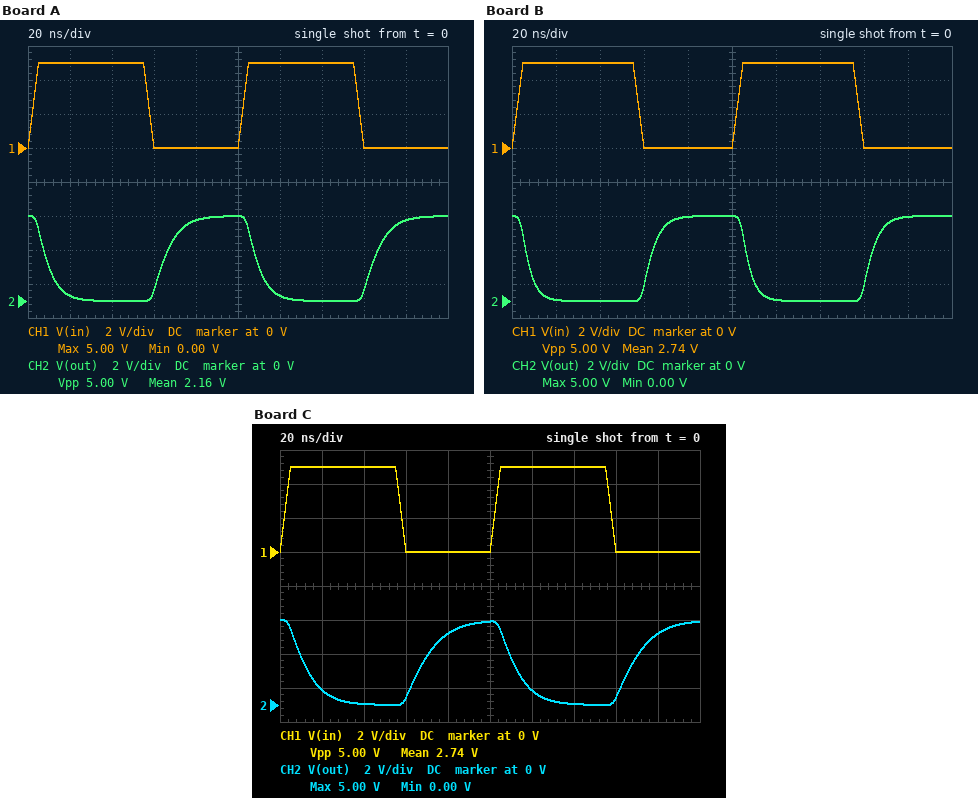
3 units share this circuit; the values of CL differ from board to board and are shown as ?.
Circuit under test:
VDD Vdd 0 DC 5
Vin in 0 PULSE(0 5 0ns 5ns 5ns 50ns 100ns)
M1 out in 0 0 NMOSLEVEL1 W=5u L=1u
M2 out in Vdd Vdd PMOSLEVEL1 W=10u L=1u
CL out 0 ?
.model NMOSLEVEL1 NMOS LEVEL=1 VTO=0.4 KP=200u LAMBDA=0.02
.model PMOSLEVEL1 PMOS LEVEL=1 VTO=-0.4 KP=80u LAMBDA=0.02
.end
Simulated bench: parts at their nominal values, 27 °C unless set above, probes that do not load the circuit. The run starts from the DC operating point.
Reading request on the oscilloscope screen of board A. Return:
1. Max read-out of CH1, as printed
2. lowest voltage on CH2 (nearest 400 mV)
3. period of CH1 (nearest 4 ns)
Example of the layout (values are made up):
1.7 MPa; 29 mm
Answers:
5.00 V; 0 V; 100 ns
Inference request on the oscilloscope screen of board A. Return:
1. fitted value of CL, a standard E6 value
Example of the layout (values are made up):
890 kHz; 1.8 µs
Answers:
22 pF
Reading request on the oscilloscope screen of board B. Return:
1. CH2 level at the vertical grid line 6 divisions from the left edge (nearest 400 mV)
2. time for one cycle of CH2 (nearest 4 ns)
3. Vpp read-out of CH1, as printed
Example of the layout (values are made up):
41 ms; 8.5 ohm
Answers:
0 V; 100 ns; 5.00 V
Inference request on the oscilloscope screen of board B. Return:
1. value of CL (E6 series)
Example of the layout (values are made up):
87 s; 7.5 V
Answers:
15 pF
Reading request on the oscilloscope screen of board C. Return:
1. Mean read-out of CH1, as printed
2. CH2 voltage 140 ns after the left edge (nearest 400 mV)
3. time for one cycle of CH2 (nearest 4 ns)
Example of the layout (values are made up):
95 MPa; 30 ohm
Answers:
2.74 V; 0 V; 100 ns
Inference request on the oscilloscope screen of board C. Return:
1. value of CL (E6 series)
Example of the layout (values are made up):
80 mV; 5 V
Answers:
33 pF
